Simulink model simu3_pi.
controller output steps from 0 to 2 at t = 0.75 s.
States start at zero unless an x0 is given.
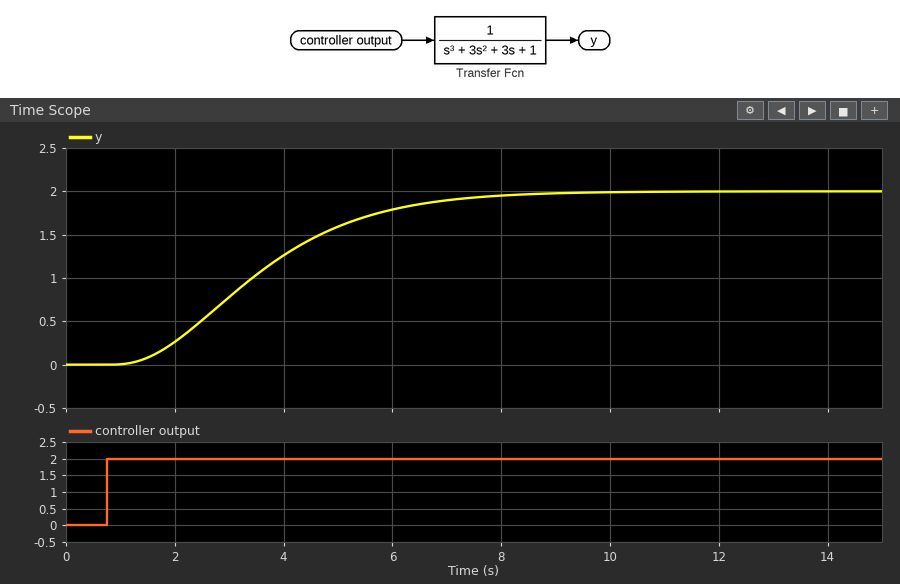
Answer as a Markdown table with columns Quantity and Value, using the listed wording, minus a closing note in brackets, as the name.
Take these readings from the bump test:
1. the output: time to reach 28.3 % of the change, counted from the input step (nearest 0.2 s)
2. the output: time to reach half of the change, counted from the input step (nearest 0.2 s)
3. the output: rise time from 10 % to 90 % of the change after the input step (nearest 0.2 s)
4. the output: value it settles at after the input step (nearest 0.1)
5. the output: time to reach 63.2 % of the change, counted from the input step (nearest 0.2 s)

| Quantity | Value |
|---|---|
| the output: time to reach 28.3 % of the change, counted from the input step | 1.8 s |
| the output: time to reach half of the change, counted from the input step | 2.6 s |
| the output: rise time from 10 % to 90 % of the change after the input step | 4.2 s |
| the output: value it settles at after the input step | 2.0 |
| the output: time to reach 63.2 % of the change, counted from the input step | 3.2 s |
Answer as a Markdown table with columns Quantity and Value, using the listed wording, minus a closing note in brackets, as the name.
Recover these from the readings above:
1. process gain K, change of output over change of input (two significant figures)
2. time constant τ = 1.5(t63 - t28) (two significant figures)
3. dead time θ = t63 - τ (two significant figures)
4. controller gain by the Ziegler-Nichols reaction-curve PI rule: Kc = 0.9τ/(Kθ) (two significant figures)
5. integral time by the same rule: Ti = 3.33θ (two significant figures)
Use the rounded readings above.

| Quantity | Value |
|---|---|
| process gain K, change of output over change of input | 1.0 |
| time constant τ = 1.5(t63 - t28) | 2.1 s |
| dead time θ = t63 - τ | 1.1 s |
| controller gain by the Ziegler-Nichols reaction-curve PI rule: Kc = 0.9τ/(Kθ) | 1.7 |
| integral time by the same rule: Ti = 3.33θ | 3.7 s |
